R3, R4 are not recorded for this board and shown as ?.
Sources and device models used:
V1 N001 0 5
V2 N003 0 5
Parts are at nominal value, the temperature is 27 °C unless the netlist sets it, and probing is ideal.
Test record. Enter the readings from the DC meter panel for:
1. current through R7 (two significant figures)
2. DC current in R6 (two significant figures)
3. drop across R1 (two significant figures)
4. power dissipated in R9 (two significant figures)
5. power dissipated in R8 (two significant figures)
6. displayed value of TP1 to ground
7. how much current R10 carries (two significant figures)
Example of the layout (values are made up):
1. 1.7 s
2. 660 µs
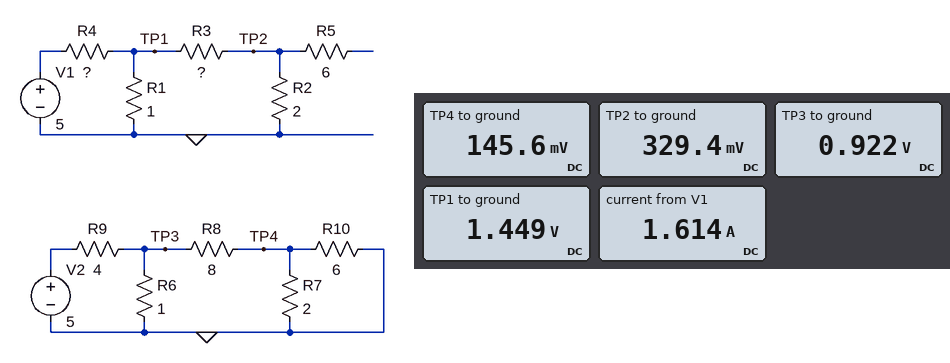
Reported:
1. 73 mA
2. 920 mA
3. 1.4 V
4. 4.2 W
5. 75 mW
6. 1.449 V
7. 24 mA
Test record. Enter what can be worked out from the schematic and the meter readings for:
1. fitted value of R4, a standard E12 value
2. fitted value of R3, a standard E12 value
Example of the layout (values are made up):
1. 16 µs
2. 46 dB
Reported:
1. 2.2 Ω
2. 6.8 Ω
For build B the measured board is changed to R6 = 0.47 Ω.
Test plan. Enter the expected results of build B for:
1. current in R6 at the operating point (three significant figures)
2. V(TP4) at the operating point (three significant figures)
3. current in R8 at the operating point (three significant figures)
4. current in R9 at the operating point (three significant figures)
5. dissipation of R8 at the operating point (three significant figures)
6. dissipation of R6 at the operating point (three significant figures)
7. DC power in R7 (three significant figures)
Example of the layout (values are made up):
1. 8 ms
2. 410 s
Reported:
1. 1.07 A
2. 79.5 mV
3. 53.0 mA
4. 1.12 A
5. 22.5 mW
6. 539 mW
7. 3.16 mW
